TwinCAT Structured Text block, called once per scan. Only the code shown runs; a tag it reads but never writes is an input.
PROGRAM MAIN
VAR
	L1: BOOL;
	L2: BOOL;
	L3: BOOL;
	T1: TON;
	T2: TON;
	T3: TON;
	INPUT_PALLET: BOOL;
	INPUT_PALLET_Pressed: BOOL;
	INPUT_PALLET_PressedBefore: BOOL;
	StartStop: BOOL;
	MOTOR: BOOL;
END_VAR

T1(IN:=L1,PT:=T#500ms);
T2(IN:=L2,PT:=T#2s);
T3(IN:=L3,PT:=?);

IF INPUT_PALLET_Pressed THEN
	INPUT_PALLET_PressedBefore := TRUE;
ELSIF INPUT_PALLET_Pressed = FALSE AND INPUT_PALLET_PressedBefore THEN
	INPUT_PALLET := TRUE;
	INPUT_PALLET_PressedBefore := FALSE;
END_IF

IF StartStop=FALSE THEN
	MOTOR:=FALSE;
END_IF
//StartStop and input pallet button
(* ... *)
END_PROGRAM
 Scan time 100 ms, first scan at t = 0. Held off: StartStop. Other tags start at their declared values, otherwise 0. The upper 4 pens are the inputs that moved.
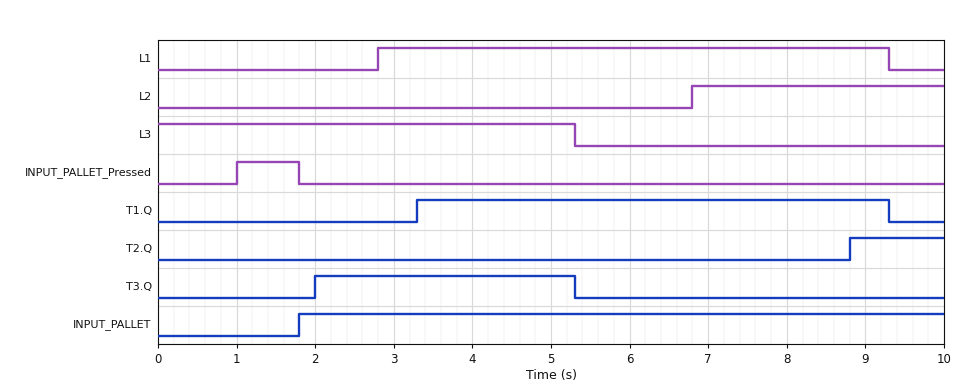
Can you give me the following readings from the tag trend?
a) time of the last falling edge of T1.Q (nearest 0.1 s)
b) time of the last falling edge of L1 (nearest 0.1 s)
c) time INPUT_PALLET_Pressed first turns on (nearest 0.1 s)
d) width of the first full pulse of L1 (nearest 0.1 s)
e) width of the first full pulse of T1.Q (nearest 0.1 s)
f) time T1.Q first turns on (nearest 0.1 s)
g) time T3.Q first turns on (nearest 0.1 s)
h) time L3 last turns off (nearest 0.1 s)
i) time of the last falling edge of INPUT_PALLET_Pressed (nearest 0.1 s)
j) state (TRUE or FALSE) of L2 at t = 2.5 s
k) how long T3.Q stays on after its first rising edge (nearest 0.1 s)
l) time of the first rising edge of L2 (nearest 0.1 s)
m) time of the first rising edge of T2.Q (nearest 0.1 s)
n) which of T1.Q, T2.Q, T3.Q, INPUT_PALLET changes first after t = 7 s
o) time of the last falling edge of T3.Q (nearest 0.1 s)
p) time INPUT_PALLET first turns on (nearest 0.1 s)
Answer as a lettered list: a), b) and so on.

a) 9.3 s
b) 9.3 s
c) 1.0 s
d) 6.5 s
e) 6.0 s
f) 3.3 s
g) 2.0 s
h) 5.3 s
i) 1.8 s
j) FALSE
k) 3.3 s
l) 6.8 s
m) 8.8 s
n) T2.Q
o) 5.3 s
p) 1.8 s
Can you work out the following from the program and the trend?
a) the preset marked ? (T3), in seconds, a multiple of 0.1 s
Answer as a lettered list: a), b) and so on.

a) 2.0 s
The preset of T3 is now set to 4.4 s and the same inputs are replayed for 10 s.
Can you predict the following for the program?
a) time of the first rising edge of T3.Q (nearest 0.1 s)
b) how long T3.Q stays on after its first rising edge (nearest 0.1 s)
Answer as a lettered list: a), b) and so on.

a) 4.4 s
b) 0.9 s
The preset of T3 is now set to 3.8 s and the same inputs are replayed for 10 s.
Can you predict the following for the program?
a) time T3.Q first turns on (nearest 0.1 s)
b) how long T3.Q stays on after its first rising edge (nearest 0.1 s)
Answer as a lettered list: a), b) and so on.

a) 3.8 s
b) 1.5 s
